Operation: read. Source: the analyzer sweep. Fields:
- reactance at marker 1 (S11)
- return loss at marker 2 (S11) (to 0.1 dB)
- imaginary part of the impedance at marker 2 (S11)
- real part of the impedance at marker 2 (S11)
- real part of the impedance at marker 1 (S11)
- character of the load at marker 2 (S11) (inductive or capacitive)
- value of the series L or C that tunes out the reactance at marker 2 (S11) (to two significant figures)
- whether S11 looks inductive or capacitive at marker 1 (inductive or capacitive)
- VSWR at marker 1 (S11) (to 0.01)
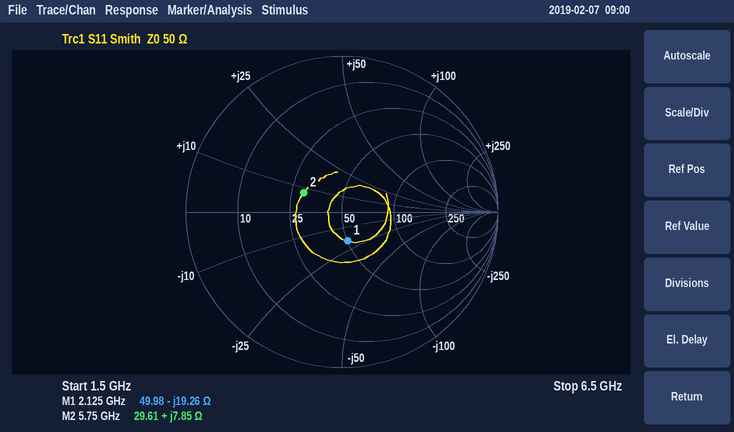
-19.26 Ω
11.3 dB
+7.85 Ω
29.61 Ω
49.98 Ω
inductive
3.5 pF
capacitive
1.47
